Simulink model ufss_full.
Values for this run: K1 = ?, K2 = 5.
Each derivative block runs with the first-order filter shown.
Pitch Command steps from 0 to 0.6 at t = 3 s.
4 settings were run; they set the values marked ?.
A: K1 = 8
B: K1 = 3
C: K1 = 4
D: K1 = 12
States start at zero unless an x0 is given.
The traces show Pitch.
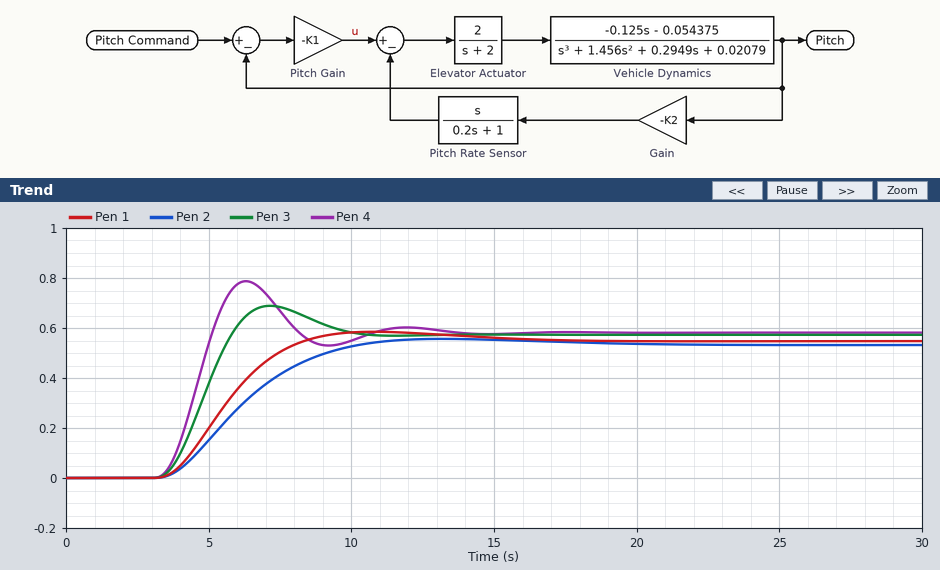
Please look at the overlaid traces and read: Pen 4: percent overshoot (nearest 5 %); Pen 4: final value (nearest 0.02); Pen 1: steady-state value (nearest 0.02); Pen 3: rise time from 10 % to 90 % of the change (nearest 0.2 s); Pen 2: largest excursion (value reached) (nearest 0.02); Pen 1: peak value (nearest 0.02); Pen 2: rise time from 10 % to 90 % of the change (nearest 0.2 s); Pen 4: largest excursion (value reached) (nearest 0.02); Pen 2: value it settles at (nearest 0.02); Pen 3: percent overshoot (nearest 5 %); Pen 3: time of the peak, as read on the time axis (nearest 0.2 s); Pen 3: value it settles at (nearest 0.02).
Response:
35 %
0.58
0.54
1.8 s
0.56
0.58
4.4 s
0.78
0.54
20 %
7.2 s
0.58
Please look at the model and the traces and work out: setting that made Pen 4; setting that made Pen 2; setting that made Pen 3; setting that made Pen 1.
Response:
D
B
A
C
